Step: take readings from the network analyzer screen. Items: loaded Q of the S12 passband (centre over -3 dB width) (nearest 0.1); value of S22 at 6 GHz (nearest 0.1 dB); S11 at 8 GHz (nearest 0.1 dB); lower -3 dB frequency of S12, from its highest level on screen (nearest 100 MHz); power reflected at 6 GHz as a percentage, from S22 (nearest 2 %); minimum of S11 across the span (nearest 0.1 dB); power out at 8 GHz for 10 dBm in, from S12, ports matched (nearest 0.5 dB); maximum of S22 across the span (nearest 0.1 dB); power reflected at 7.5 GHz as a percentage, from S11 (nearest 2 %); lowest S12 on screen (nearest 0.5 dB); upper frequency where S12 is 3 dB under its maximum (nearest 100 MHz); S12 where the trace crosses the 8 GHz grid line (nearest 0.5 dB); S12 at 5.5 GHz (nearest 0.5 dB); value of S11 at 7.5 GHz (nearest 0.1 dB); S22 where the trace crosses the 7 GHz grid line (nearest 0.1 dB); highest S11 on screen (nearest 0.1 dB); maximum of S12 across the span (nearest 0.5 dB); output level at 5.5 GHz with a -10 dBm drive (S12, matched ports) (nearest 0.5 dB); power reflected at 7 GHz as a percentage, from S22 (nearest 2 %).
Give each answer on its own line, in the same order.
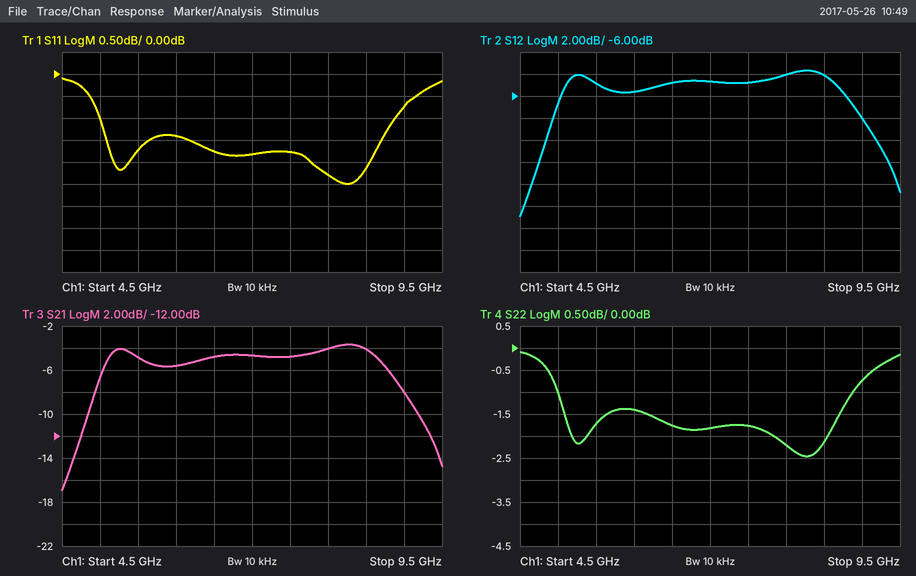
1.8
-1.4 dB
-2.3 dB
5.0 GHz
72 %
-2.5 dB
6.0 dBm
-0.1 dB
66 %
-17.0 dB
8.9 GHz
-4.0 dB
-5.0 dB
-1.8 dB
-1.8 dB
-0.1 dB
-3.5 dB
-15.0 dBm
66 %
